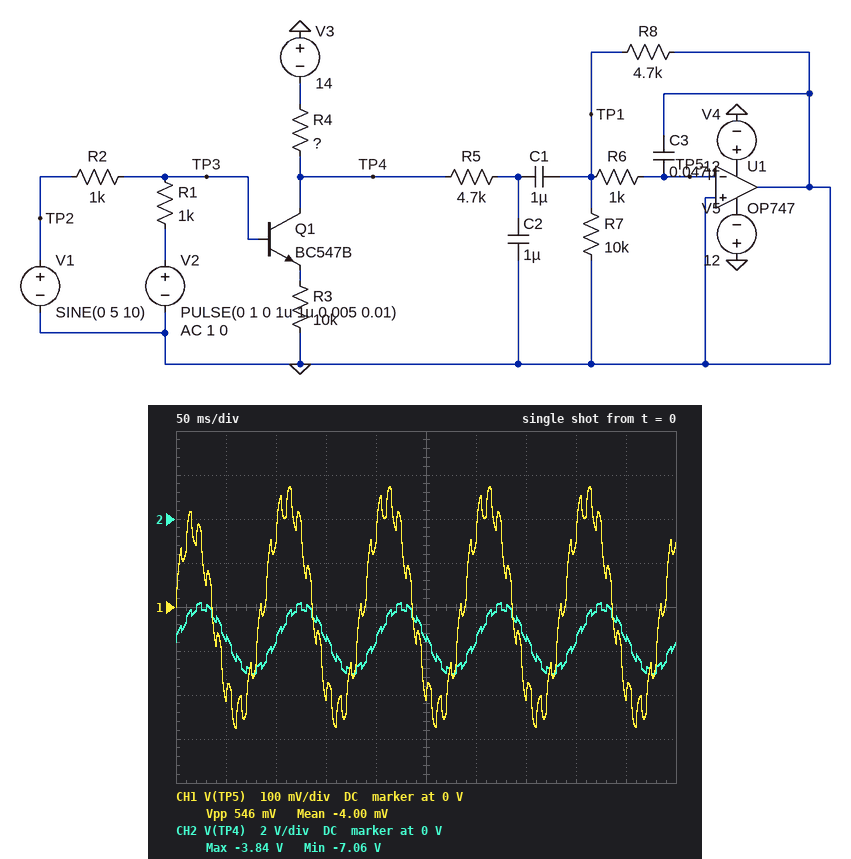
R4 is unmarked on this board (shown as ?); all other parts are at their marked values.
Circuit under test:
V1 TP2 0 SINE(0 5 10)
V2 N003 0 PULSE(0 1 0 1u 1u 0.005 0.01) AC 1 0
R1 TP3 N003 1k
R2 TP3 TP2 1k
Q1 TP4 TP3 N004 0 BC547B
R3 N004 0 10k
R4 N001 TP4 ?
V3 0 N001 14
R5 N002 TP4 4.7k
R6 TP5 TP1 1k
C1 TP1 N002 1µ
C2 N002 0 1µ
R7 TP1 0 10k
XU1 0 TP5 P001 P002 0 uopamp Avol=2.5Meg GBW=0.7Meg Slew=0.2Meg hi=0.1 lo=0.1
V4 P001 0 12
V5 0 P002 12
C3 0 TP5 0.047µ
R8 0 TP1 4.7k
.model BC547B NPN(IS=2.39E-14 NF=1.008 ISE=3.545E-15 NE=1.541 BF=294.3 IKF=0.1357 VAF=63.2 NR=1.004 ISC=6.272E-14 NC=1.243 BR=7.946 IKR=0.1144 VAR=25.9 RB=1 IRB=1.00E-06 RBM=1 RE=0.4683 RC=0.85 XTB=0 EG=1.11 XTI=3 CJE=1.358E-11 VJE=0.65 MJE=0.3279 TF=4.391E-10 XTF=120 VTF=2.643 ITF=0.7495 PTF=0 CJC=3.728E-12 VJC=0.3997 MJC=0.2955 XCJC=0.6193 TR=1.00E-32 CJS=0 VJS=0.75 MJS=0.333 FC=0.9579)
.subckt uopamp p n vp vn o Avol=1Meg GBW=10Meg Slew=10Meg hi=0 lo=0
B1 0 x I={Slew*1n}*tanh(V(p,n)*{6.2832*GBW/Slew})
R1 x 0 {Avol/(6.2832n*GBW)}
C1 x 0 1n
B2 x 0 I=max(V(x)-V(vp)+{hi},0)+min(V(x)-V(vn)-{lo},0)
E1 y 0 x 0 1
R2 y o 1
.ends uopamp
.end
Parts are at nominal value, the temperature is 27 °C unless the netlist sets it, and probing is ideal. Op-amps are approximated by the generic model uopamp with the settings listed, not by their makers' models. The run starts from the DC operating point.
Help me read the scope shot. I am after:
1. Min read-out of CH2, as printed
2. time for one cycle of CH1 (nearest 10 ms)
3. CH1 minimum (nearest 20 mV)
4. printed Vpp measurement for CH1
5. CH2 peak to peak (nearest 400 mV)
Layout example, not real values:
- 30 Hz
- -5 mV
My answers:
- -7.06 V
- 100 ms
- -280 mV
- 546 mV
- 3.2 V
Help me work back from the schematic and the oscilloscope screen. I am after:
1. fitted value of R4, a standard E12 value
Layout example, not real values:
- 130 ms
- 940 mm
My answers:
- 820 Ω
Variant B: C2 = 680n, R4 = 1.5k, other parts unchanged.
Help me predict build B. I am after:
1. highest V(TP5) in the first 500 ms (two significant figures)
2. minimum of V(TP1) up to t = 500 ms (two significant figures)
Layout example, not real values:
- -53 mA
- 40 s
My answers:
- 340 mV
- -350 mV
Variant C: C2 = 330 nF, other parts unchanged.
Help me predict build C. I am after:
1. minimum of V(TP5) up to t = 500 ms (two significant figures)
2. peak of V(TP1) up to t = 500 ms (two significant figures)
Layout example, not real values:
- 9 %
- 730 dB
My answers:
- -310 mV
- 310 mV
